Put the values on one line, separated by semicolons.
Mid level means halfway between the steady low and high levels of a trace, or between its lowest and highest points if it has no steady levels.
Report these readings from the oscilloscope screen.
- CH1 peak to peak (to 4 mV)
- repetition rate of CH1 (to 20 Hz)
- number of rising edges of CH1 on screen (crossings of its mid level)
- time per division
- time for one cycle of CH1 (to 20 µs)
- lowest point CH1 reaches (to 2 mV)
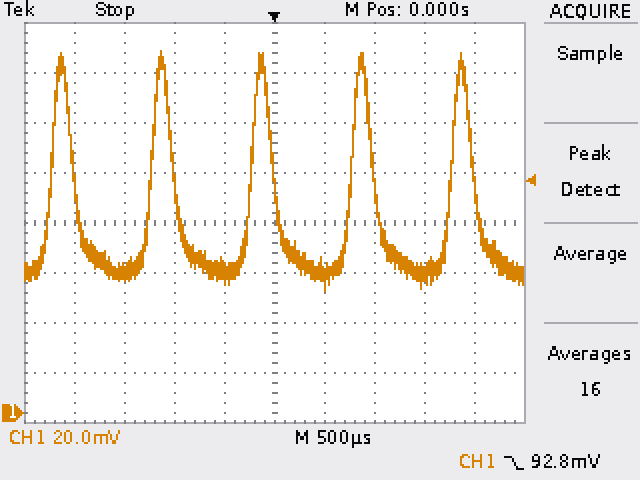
96 mV; 1.00 kHz; 5; 500 µs; 1.00 ms; 48 mV
